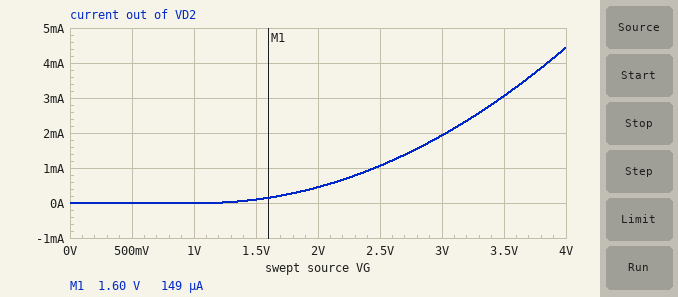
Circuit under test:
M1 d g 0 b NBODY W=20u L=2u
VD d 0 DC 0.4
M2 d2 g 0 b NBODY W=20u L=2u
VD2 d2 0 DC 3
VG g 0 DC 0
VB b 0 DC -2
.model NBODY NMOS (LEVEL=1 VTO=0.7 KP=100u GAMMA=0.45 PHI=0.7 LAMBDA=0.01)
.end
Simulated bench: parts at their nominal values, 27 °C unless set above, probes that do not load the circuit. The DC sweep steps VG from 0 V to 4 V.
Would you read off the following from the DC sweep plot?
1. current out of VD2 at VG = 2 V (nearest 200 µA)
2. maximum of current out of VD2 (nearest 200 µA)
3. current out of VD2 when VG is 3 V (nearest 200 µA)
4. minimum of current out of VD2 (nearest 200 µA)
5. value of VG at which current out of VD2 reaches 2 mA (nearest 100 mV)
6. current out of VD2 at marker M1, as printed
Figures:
400 µA
4.4 mA
2.0 mA
0 A
3.0 V
149 µA
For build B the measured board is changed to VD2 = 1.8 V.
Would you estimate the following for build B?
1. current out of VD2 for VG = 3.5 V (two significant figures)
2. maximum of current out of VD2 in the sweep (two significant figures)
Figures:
2.8 mA
3.7 mA
